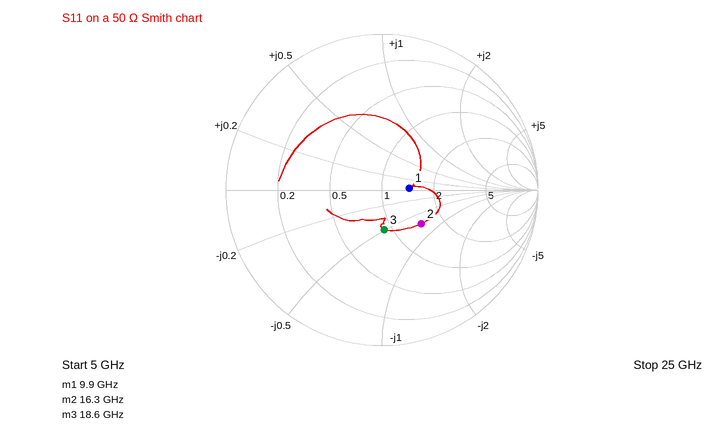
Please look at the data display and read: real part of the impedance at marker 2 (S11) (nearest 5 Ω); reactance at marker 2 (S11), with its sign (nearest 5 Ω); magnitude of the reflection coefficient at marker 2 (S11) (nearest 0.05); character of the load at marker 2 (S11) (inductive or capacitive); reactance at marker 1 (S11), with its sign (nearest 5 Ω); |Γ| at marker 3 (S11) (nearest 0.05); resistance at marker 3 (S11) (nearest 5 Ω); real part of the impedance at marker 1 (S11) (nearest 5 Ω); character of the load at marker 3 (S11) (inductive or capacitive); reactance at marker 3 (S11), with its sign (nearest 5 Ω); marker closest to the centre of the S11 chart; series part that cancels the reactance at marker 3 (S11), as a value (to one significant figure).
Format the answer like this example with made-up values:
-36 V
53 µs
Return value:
75 Ω
-35 Ω
0.35
capacitive
0 Ω
0.25
45 Ω
70 Ω
capacitive
-25 Ω
marker 1
200 pH
